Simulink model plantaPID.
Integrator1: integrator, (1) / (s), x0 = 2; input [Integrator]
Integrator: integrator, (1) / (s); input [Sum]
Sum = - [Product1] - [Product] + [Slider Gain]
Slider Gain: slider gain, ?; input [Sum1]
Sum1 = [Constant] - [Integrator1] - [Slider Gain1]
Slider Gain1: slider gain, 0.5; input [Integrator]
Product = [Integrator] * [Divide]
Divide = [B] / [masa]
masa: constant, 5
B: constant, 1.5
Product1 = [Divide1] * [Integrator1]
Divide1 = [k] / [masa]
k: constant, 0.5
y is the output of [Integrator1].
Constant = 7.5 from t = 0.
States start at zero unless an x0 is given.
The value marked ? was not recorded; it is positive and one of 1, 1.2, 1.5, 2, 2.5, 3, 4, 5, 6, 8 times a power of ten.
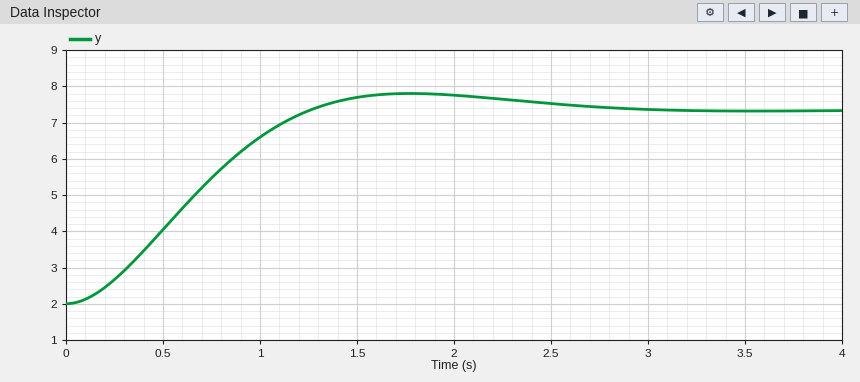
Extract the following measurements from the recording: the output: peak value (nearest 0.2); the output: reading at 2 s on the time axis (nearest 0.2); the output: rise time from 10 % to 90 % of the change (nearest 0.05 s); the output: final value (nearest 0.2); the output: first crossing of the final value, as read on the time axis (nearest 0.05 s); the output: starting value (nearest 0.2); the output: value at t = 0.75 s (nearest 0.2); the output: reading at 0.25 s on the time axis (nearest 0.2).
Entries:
7.8
7.8
0.85 s
7.4
1.25 s
2.0
5.4
2.6
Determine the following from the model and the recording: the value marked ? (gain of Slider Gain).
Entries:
5
